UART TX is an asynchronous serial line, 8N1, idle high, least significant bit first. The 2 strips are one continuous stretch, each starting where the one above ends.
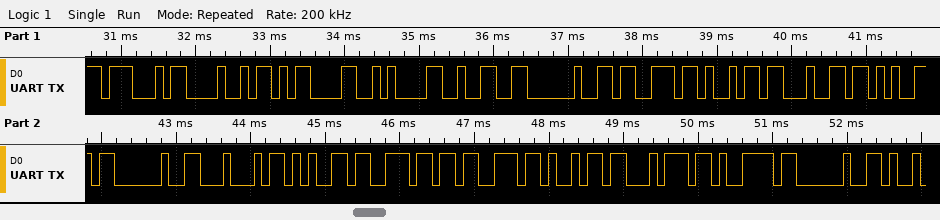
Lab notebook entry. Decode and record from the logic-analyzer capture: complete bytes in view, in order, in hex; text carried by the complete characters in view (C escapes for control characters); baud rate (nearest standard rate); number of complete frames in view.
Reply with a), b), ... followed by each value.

a) 47 48 0D 0A 32 20 73 69 64 65 20 44 65 6E 73 69 74 79 20
b) "GH\r\n2 side Density "
c) 9600 baud
d) 19
